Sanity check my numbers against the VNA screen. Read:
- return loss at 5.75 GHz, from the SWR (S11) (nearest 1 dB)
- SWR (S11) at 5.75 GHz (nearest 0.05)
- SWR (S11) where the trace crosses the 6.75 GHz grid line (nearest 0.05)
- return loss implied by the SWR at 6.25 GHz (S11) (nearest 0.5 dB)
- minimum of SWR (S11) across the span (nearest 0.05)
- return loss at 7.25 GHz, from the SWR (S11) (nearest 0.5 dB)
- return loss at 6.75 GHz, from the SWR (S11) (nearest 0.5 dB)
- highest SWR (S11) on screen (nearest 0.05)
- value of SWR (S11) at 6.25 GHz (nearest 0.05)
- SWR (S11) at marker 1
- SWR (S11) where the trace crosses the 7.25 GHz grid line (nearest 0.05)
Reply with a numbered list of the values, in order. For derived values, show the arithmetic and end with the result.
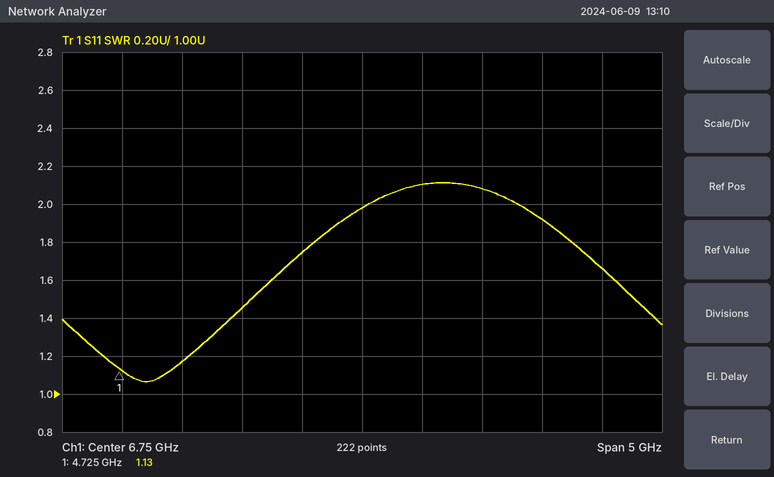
1. −20 log10((1.45 − 1)/(1.45 + 1)) ≈ 15 dB
2. 1.45
3. 2.00
4. −20 log10((1.75 − 1)/(1.75 + 1)) ≈ 11.3 dB, so 11.5 dB to the nearest 0.5 dB
5. 1.05
6. −20 log10((2.1 − 1)/(2.1 + 1)) ≈ 9.0 dB
7. −20 log10((2 − 1)/(2 + 1)) ≈ 9.5 dB
8. 2.10
9. 1.75
10. 1.13
11. 2.10
